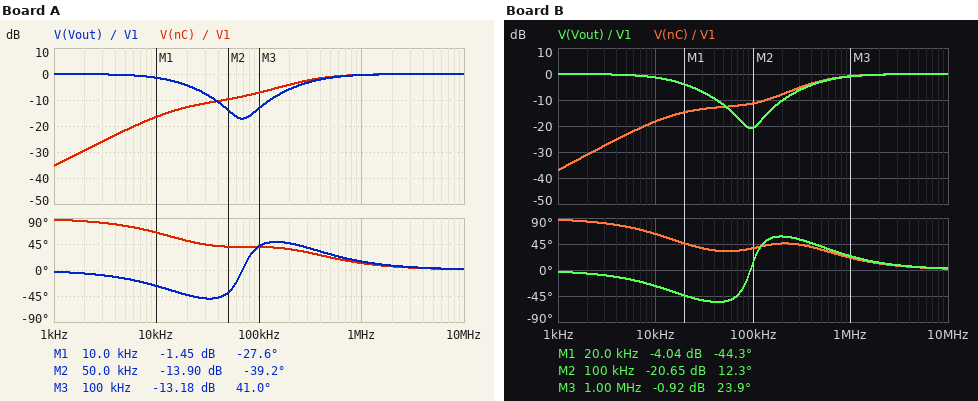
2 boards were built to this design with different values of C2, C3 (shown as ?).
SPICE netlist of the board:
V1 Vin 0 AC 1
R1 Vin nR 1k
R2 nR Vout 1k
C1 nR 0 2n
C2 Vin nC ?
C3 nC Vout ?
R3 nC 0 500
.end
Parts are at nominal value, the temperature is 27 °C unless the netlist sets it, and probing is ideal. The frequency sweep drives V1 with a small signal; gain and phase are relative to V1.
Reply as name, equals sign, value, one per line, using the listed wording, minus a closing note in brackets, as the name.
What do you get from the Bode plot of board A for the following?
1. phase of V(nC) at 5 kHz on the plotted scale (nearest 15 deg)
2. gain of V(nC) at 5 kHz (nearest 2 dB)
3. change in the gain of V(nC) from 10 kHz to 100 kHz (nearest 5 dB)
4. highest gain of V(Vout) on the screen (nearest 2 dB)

phase of V(nC) at 5 kHz on the plotted scale = 75 deg
gain of V(nC) at 5 kHz = -22 dB
change in the gain of V(nC) from 10 kHz to 100 kHz = 10 dB
highest gain of V(Vout) on the screen = 0 dB
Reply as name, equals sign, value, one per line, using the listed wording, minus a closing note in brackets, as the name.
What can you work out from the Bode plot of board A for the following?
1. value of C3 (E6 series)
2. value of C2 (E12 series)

value of C3 = 3.3 nF
value of C2 = 2.2 nF
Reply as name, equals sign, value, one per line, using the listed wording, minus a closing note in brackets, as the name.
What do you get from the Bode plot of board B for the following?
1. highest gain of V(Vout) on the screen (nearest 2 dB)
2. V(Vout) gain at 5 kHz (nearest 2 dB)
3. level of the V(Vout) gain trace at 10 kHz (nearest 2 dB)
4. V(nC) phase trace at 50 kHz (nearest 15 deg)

highest gain of V(Vout) on the screen = 0 dB
V(Vout) gain at 5 kHz = 0 dB
level of the V(Vout) gain trace at 10 kHz = -2 dB
V(nC) phase trace at 50 kHz = 30 deg
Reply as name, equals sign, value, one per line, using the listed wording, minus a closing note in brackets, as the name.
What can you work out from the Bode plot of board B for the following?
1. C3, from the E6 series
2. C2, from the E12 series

C3, from the E6 series = 3.3 nF
C2, from the E12 series = 1.2 nF
